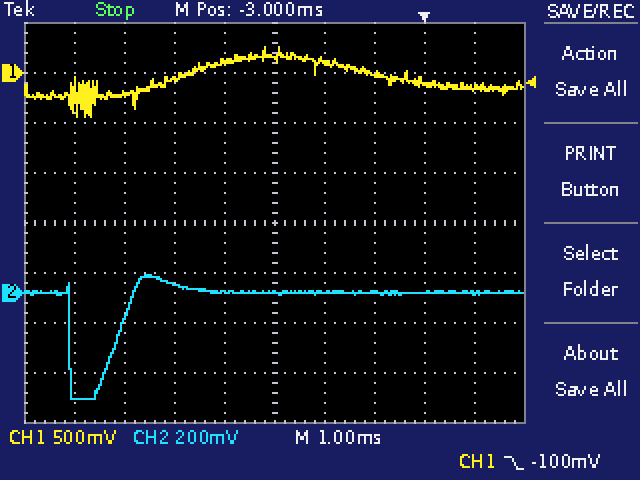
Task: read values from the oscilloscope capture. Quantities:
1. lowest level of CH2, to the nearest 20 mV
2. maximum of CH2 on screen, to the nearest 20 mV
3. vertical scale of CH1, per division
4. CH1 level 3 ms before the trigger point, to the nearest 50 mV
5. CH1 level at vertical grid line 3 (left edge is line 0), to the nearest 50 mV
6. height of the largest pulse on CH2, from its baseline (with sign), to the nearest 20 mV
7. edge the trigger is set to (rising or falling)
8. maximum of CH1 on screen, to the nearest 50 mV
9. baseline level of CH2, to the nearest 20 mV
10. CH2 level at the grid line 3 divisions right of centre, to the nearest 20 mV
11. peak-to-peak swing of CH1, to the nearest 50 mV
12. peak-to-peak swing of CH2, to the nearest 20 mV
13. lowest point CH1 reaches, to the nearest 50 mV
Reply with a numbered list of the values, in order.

1. -420 mV
2. 80 mV
3. 500 mV
4. 150 mV
5. -50 mV
6. -420 mV
7. falling
8. 250 mV
9. 0 mV
10. 0 mV
11. 700 mV
12. 500 mV
13. -450 mV
